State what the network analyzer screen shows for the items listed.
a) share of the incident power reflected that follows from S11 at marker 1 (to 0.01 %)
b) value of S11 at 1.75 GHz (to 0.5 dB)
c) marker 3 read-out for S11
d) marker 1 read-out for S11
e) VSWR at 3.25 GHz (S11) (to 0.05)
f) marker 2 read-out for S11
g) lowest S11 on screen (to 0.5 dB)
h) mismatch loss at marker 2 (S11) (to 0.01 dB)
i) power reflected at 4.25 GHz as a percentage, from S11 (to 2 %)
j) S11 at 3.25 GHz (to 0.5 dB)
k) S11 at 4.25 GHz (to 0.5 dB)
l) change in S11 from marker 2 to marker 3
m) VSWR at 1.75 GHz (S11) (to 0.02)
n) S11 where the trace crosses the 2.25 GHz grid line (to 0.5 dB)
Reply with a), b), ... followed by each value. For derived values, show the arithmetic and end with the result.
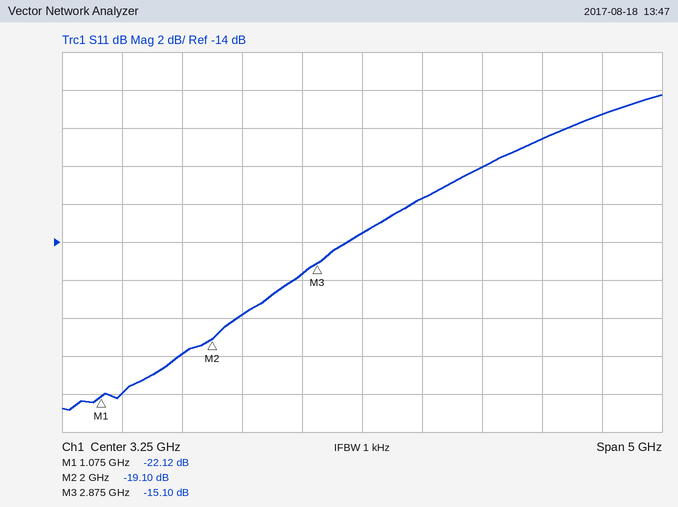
a) 10^(-22.12/10) ≈ 0.61 %
b) -20.0 dB
c) -15.10 dB
d) -22.12 dB
e) |Γ| = 10^(-13.5/20) = 0.2113; VSWR = (1 + 0.2113)/(1 − 0.2113) ≈ 1.54, so 1.55 to the nearest 0.05
f) -19.10 dB
g) -23.0 dB
h) −10 log10(1 − 10^(-19.1/10)) ≈ 0.05 dB
i) 10^(-10/10) ≈ 10 %
j) -13.5 dB
k) -10.0 dB
l) -15.1 − (-19.1) = 4.00 dB
m) |Γ| = 10^(-20/20) = 0.1000; VSWR = (1 + 0.1000)/(1 − 0.1000) ≈ 1.22
n) -18.0 dB
